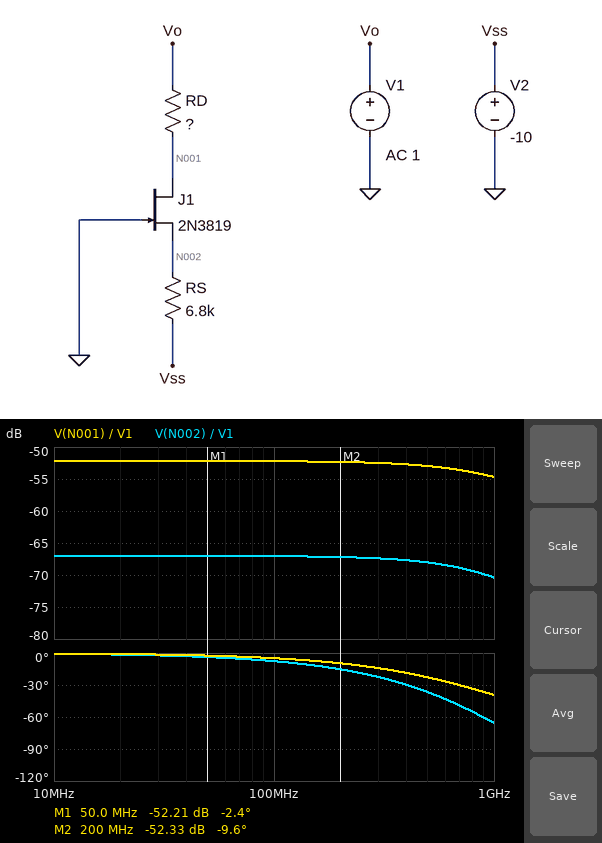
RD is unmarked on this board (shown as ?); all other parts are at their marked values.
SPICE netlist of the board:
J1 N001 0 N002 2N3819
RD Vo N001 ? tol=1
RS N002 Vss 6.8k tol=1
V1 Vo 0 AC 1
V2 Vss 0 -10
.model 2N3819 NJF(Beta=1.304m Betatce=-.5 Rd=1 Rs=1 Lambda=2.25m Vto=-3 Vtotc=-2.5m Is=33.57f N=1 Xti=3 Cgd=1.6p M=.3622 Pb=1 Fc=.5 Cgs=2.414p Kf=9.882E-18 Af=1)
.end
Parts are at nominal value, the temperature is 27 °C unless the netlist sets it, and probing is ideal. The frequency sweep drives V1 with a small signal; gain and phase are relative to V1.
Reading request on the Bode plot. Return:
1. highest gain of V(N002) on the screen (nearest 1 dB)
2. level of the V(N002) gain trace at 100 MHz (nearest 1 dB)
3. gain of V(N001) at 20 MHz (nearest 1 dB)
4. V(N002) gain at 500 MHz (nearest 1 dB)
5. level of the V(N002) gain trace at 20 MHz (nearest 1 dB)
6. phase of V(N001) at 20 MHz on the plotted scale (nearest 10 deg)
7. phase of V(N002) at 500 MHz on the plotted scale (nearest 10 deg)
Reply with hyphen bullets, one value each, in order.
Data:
- -67 dB
- -67 dB
- -52 dB
- -68 dB
- -67 dB
- 0 deg
- -40 deg
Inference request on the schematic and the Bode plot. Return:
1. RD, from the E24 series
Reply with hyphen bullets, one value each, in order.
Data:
- 22 kΩ
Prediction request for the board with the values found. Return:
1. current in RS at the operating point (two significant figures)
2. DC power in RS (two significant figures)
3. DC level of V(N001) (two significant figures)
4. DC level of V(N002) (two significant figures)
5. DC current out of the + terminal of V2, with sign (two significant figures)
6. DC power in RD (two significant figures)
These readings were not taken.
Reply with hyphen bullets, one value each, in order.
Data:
- 1.4 mA
- 13 mW
- -590 mV
- -630 mV
- -1.4 mA
- 16 µW
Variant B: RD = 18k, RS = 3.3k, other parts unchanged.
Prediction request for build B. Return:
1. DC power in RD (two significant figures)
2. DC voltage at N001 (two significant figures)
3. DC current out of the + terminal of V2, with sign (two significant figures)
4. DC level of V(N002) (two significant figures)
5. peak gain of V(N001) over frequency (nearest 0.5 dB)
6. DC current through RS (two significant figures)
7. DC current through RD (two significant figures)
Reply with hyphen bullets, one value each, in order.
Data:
- 20 µW
- -600 mV
- -2.8 mA
- -650 mV
- -52.5 dB
- 2.8 mA
- 33 µA
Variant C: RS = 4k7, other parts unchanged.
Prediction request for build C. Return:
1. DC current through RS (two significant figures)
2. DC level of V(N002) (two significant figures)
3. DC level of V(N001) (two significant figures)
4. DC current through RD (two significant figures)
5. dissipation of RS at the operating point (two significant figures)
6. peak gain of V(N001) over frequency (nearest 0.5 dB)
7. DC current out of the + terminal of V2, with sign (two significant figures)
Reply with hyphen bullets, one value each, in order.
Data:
- 2.0 mA
- -640 mV
- -600 mV
- 27 µA
- 19 mW
- -53.5 dB
- -2.0 mA
